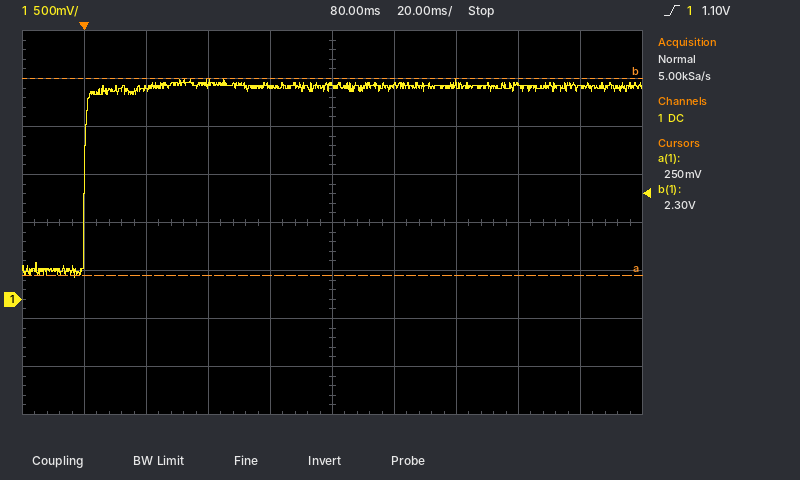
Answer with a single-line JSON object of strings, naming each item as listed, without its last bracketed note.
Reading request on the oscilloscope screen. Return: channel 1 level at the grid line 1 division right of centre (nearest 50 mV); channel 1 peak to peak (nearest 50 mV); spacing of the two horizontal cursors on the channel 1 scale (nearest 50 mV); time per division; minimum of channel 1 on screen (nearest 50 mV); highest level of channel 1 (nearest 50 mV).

{"channel 1 level at the grid line 1 division right of centre": "2.25 V", "channel 1 peak to peak": "2.05 V", "spacing of the two horizontal cursors on the channel 1 scale": "2.05 V", "time per division": "20 ms", "minimum of channel 1 on screen": "250 mV", "highest level of channel 1": "2.30 V"}
